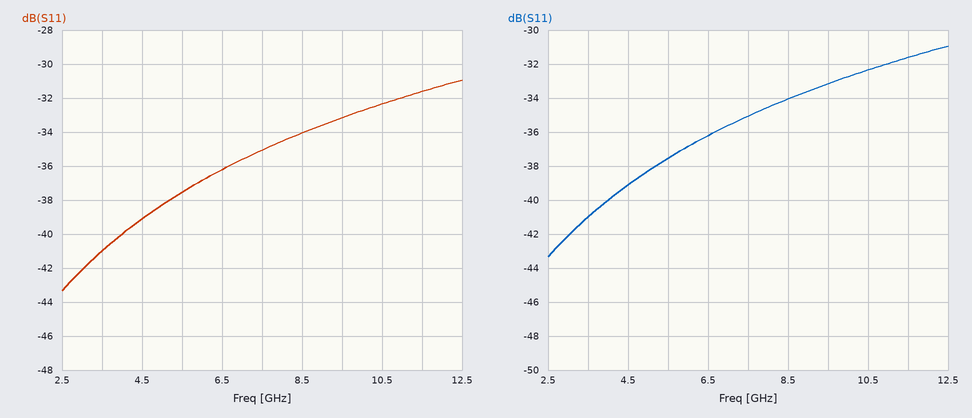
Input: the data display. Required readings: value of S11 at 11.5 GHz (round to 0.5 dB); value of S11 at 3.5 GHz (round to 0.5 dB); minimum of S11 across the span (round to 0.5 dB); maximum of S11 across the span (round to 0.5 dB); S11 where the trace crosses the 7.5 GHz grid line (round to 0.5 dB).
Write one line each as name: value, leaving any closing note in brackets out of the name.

value of S11 at 11.5 GHz: -31.5 dB
value of S11 at 3.5 GHz: -41.0 dB
minimum of S11 across the span: -43.5 dB
maximum of S11 across the span: -31.0 dB
S11 where the trace crosses the 7.5 GHz grid line: -35.0 dB
